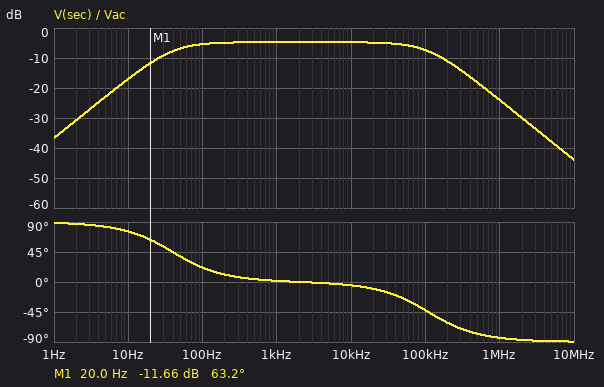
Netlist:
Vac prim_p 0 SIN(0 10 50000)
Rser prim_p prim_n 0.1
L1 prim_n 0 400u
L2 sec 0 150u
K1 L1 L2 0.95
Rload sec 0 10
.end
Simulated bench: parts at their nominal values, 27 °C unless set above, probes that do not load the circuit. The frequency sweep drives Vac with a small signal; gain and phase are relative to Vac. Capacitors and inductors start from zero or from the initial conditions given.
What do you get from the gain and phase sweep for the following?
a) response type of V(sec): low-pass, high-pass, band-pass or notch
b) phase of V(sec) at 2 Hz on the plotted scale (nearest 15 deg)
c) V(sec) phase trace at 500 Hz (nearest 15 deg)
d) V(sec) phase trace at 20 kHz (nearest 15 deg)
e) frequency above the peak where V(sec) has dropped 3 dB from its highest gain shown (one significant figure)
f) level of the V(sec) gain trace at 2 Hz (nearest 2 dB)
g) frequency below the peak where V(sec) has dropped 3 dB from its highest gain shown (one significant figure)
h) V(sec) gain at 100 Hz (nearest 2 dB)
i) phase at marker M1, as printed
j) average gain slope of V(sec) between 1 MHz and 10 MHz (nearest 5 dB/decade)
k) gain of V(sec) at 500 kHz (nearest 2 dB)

band-pass
90 deg
0 deg
-15 deg
100 kHz
-30 dB
40 Hz
-6 dB
63.2 deg
-20 dB/decade
-18 dB
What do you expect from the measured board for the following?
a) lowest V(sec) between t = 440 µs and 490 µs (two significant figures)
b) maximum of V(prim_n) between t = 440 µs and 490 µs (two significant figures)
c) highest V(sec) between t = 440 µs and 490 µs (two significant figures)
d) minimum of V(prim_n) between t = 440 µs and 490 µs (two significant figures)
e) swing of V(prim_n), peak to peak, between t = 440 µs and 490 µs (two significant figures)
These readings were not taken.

-5.3 V
10 V
5.3 V
-10 V
20 V
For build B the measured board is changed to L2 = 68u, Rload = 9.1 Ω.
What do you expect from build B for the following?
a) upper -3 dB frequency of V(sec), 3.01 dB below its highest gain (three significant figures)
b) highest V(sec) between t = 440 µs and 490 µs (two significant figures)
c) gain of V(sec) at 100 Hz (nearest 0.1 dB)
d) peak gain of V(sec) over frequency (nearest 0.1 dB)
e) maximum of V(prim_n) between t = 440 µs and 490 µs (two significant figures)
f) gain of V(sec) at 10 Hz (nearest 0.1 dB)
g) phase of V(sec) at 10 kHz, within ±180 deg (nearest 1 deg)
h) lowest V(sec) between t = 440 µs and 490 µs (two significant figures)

219 kHz
3.8 V
-8.8 dB
-8.2 dB
10 V
-20.4 dB
-2 deg
-3.8 V
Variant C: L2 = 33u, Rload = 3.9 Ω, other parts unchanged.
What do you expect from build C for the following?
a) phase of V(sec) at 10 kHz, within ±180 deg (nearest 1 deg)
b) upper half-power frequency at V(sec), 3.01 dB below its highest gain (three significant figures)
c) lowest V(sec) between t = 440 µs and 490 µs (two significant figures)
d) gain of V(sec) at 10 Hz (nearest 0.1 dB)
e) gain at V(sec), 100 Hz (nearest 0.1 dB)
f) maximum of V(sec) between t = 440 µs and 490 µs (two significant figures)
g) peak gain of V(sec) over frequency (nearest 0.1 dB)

-3 deg
193 kHz
-2.6 V
-23.5 dB
-11.9 dB
2.6 V
-11.3 dB
